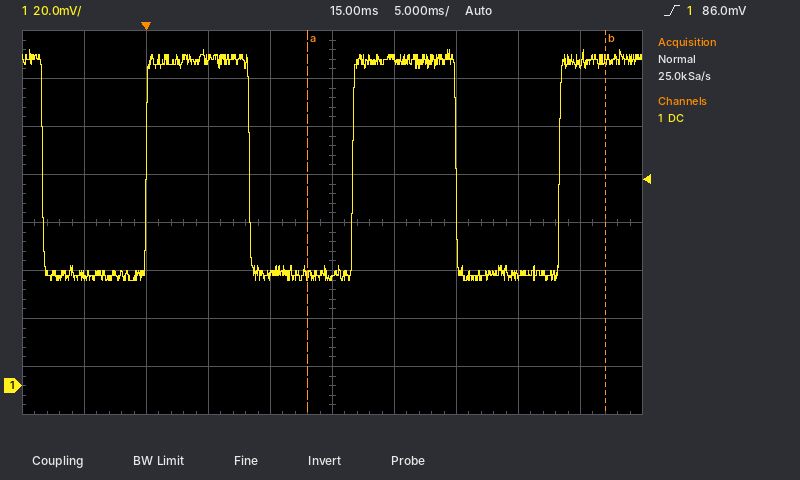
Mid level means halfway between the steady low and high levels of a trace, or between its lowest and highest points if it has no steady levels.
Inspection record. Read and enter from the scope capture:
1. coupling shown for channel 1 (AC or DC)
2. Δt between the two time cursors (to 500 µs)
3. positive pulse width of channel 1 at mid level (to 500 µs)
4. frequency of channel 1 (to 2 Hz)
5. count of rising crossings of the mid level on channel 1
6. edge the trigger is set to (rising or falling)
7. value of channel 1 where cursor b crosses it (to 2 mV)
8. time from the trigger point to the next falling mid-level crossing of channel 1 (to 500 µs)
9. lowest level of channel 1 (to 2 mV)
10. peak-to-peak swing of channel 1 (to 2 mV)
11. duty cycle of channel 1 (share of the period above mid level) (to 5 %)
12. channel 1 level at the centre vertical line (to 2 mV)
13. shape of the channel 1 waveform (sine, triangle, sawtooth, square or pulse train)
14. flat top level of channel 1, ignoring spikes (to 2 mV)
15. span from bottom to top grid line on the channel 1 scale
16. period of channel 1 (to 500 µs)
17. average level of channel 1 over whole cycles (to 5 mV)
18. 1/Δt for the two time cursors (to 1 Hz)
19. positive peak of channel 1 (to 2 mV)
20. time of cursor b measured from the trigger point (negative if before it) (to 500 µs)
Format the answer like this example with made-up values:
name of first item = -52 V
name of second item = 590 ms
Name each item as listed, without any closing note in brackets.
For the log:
coupling shown for channel 1 = DC
Δt between the two time cursors = 24.0 ms
positive pulse width of channel 1 at mid level = 8.5 ms
frequency of channel 1 = 60 Hz
count of rising crossings of the mid level on channel 1 = 3
edge the trigger is set to = rising
value of channel 1 where cursor b crosses it = 136 mV
time from the trigger point to the next falling mid-level crossing of channel 1 = 8.5 ms
lowest level of channel 1 = 44 mV
peak-to-peak swing of channel 1 = 96 mV
duty cycle of channel 1 (share of the period above mid level) = 50 %
channel 1 level at the centre vertical line = 46 mV
shape of the channel 1 waveform = square
flat top level of channel 1, ignoring spikes = 136 mV
span from bottom to top grid line on the channel 1 scale = 160 mV
period of channel 1 = 16.5 ms
average level of channel 1 over whole cycles = 90 mV
1/Δt for the two time cursors = 42 Hz
positive peak of channel 1 = 140 mV
time of cursor b measured from the trigger point (negative if before it) = +37.0 ms
